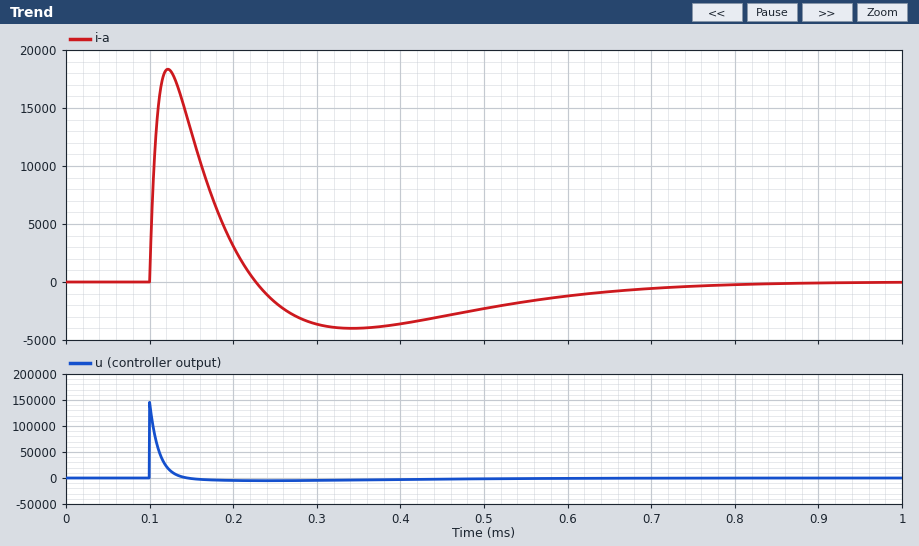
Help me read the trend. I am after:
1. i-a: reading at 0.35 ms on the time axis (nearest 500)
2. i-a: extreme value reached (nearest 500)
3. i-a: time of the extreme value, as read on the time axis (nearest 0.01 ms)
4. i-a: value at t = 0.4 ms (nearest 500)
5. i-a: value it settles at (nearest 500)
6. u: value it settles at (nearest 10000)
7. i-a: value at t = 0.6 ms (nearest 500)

-4000
18500
0.12 ms
-3500
0
0
-1000
